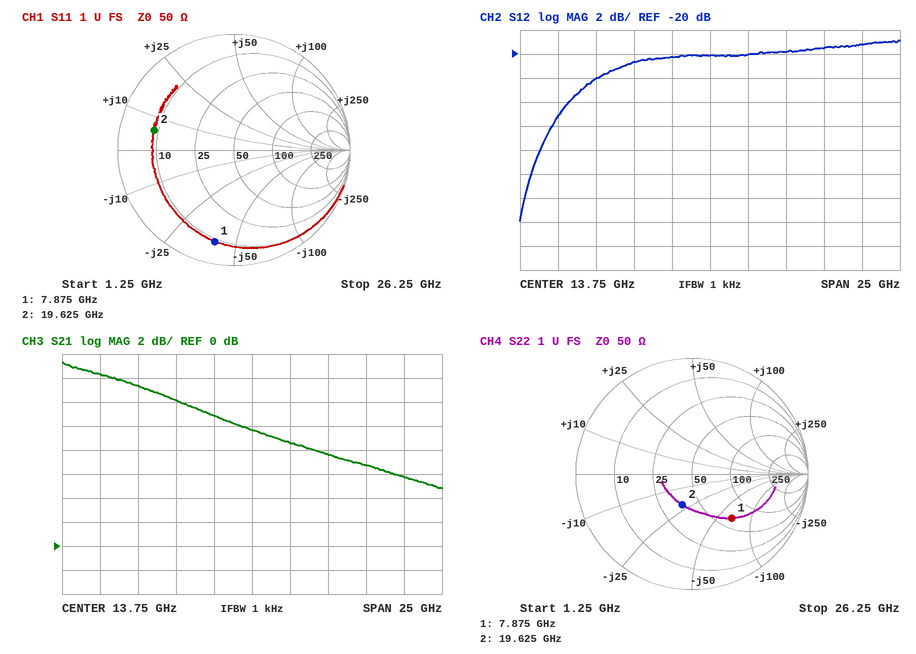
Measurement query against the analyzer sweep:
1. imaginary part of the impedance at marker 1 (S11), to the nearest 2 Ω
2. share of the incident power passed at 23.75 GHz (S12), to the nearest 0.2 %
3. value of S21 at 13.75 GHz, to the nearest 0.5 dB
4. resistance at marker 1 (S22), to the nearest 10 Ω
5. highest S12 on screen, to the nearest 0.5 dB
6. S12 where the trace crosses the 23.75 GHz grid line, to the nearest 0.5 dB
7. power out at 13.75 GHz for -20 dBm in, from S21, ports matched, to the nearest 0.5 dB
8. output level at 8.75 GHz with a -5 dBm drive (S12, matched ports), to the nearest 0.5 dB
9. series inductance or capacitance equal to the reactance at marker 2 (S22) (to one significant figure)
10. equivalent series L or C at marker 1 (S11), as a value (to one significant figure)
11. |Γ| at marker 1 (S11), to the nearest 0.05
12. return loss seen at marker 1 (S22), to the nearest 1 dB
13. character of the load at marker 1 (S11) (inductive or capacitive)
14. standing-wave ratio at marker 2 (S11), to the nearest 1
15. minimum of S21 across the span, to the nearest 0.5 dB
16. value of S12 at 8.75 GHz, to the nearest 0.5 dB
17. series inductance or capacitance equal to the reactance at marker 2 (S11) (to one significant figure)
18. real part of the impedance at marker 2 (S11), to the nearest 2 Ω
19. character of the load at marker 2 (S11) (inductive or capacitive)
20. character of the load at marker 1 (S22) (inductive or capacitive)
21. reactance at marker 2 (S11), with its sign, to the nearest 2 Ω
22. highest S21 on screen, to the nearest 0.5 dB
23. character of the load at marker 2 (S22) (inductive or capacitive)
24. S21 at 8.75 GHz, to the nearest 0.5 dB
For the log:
-40 Ω
1.2 %
9.5 dB
60 Ω
-19.0 dB
-19.0 dB
-10.5 dBm
-25.5 dBm
400 fF
500 fF
0.80
6 dB
capacitive
6
5.0 dB
-20.5 dB
50 pH
8 Ω
inductive
capacitive
+6 Ω
15.5 dB
capacitive
12.0 dB
